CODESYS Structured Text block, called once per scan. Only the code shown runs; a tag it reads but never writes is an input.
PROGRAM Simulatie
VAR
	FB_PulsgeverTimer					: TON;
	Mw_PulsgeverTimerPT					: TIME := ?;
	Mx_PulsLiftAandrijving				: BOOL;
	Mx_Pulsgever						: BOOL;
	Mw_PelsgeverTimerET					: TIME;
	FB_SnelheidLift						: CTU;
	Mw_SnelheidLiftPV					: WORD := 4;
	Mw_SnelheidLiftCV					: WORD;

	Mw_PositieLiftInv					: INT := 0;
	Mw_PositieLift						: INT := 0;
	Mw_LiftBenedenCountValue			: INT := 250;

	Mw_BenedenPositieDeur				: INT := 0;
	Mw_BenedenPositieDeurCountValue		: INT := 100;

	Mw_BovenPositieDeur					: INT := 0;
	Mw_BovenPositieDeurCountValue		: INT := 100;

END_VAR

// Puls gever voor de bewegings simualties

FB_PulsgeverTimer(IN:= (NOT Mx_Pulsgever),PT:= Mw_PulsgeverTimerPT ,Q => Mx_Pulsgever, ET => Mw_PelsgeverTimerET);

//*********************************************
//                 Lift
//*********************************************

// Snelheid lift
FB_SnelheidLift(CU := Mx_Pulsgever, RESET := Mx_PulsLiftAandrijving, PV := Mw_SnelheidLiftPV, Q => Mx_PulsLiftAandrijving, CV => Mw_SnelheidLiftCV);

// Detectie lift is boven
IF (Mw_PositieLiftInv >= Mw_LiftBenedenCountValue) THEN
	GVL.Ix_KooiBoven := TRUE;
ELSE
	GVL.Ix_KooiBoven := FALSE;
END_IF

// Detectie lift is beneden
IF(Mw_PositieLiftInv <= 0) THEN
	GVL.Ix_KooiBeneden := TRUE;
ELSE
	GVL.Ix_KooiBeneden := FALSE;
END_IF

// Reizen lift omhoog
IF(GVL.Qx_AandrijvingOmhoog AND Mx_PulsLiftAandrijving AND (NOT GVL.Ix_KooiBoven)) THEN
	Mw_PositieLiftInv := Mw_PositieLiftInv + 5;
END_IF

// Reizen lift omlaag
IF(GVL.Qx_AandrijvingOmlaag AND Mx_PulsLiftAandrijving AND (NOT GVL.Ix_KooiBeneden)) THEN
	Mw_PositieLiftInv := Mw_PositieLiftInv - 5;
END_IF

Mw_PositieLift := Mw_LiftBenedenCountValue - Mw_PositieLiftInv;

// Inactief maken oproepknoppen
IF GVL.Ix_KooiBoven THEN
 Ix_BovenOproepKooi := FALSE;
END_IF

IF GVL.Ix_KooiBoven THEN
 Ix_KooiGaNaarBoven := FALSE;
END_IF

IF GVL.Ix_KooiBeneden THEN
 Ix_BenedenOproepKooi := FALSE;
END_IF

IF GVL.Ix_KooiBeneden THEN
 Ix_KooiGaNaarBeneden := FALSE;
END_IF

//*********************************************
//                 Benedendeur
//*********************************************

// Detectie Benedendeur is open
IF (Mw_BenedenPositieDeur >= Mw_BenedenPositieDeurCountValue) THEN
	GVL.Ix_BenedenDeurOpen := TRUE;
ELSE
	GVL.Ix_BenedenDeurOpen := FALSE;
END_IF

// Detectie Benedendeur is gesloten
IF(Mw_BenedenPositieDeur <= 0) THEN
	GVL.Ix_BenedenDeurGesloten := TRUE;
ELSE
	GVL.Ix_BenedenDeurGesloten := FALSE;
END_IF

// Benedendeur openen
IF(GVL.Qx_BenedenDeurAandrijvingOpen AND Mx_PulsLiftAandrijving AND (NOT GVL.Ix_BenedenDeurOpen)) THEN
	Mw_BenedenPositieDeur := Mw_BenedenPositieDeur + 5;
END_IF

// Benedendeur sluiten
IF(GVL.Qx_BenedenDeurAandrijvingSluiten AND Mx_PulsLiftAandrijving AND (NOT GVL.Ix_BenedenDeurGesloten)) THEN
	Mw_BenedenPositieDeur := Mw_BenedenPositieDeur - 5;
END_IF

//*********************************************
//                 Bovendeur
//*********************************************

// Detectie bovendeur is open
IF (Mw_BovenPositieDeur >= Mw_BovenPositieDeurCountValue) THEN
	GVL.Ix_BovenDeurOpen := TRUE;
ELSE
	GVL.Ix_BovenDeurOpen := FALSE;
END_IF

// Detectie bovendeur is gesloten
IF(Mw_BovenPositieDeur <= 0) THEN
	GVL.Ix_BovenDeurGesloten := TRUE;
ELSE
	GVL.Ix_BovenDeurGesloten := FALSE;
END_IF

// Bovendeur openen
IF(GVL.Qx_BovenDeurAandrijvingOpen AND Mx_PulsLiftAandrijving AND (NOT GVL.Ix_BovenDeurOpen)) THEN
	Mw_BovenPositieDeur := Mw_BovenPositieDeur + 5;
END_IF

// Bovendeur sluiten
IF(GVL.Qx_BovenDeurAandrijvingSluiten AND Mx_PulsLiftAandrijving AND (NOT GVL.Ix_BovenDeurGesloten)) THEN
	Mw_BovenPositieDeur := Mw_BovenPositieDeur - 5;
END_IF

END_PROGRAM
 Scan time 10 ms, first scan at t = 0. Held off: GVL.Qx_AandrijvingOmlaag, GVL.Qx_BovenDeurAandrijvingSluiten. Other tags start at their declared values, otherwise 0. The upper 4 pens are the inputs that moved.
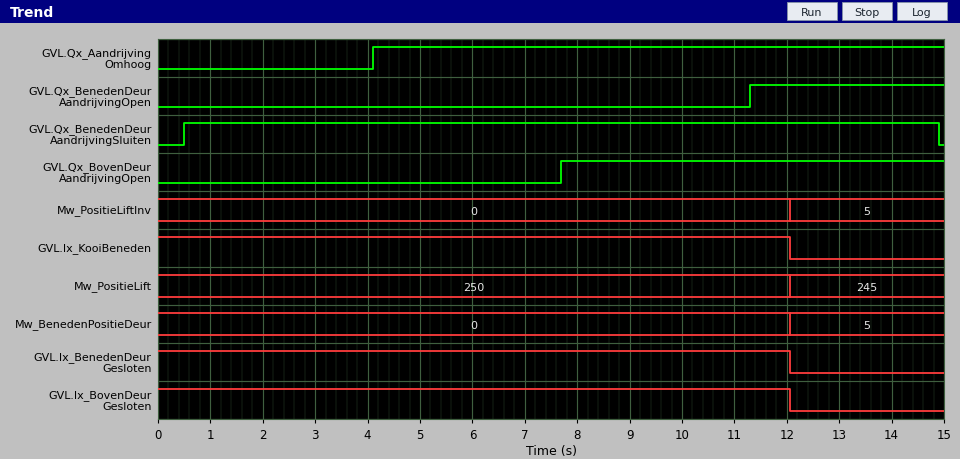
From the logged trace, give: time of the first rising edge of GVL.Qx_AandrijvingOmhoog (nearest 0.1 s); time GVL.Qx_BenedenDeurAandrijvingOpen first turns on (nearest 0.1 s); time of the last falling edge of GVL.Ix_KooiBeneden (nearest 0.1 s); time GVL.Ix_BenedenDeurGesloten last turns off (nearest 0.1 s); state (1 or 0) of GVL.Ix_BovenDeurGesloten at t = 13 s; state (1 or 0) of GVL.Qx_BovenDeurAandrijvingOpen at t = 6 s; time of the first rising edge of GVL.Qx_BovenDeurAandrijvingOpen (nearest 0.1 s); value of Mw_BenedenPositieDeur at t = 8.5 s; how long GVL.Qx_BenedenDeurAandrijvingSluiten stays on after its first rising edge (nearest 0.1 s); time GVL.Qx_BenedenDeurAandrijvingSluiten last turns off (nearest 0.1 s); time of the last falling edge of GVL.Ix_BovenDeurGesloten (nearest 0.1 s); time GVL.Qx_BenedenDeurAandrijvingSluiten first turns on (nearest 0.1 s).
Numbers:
4.1 s
11.3 s
12.1 s
12.1 s
0
0
7.7 s
0
14.4 s
14.9 s
12.1 s
0.5 s
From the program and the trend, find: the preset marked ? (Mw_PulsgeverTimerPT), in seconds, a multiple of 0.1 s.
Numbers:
3.0 s
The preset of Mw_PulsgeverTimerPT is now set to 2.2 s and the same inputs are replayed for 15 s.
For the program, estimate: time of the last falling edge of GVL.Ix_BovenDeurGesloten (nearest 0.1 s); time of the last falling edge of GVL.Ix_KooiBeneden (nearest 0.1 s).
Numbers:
8.9 s
8.9 s
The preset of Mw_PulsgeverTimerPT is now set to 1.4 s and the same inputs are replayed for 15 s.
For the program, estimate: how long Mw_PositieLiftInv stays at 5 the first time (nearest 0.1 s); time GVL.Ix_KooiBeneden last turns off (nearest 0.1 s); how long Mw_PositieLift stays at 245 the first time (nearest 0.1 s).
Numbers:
5.7 s
5.7 s
5.7 s
